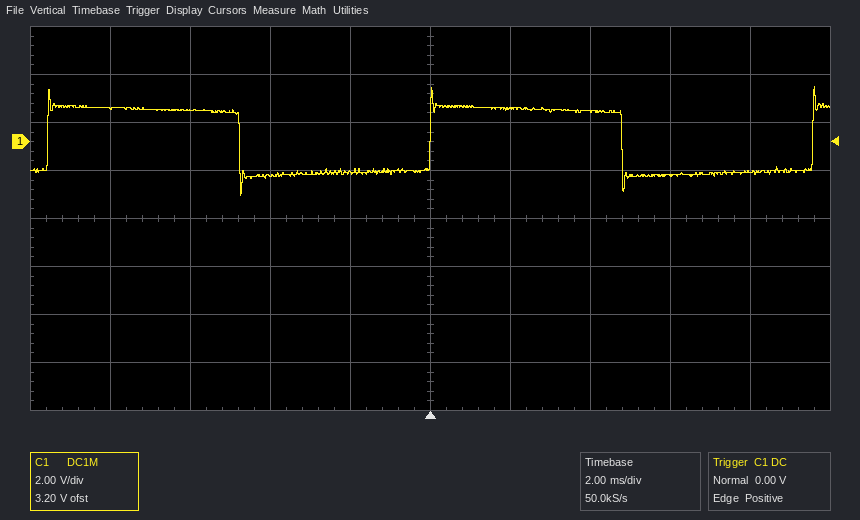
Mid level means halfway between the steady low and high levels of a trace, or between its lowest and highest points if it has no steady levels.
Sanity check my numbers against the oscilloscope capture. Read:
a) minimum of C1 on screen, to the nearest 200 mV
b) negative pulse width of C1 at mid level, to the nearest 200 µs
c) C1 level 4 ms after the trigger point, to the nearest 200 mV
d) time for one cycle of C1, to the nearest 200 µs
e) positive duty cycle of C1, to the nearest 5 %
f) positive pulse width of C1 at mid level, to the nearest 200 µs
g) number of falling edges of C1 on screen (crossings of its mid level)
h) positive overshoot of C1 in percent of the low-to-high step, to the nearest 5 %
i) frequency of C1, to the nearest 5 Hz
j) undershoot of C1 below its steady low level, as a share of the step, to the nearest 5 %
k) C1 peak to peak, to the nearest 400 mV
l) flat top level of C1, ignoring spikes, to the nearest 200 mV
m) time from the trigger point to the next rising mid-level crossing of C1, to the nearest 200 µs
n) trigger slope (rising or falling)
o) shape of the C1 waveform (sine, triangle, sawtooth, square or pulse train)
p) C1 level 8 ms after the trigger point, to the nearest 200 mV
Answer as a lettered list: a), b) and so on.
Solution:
a) -2.2 V
b) 4.8 ms
c) 1.2 V
d) 9.6 ms
e) 50 %
f) 4.8 ms
g) 2
h) 35 %
i) 105 Hz
j) 35 %
k) 4.4 V
l) 1.4 V
m) 9.6 ms
n) rising
o) square
p) -1.2 V
